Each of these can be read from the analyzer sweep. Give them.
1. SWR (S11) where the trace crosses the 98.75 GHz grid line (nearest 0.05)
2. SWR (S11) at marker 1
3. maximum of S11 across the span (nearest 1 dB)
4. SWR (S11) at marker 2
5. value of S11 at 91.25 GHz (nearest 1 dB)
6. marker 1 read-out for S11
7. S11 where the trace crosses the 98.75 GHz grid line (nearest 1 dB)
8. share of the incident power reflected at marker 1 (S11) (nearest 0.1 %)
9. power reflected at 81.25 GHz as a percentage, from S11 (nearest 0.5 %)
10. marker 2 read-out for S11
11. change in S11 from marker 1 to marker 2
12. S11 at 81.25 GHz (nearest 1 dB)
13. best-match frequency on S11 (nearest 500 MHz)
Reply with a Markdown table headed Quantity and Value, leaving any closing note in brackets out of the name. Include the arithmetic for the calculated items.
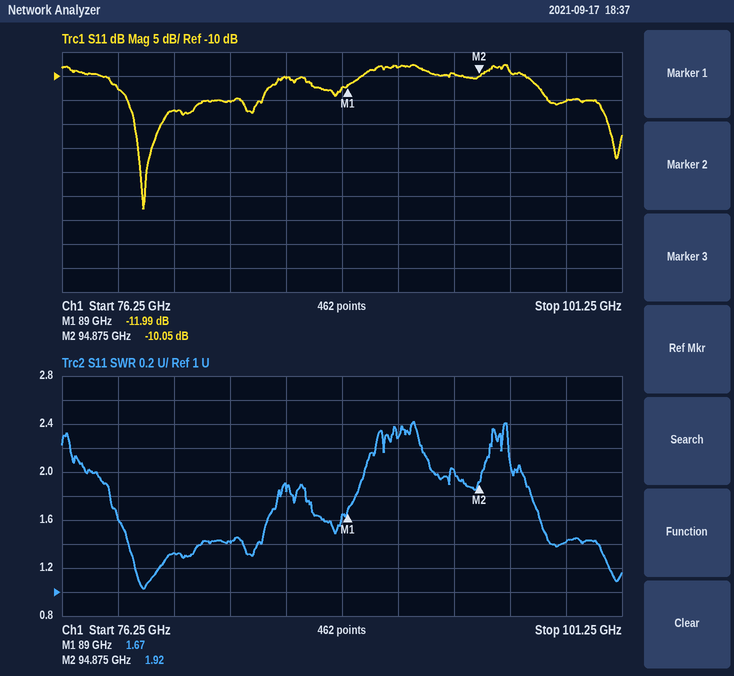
| Quantity | Value |
|---|---|
| SWR (S11) where the trace crosses the 98.75 GHz grid line | 1.40 |
| SWR (S11) at marker 1 | 1.67 |
| maximum of S11 across the span | -8 dB |
| SWR (S11) at marker 2 | 1.92 |
| value of S11 at 91.25 GHz | -8 dB |
| marker 1 read-out for S11 | -11.99 dB |
| S11 where the trace crosses the 98.75 GHz grid line | -15 dB |
| share of the incident power reflected at marker 1 (S11) | 10^(-11.99/10) ≈ 6.3 % |
| power reflected at 81.25 GHz as a percentage, from S11 | 10^(-17/10) ≈ 2.0 % |
| marker 2 read-out for S11 | -10.05 dB |
| change in S11 from marker 1 to marker 2 | -10.05 − (-11.99) = 1.94 dB |
| S11 at 81.25 GHz | -17 dB |
| best-match frequency on S11 | 80.0 GHz |
